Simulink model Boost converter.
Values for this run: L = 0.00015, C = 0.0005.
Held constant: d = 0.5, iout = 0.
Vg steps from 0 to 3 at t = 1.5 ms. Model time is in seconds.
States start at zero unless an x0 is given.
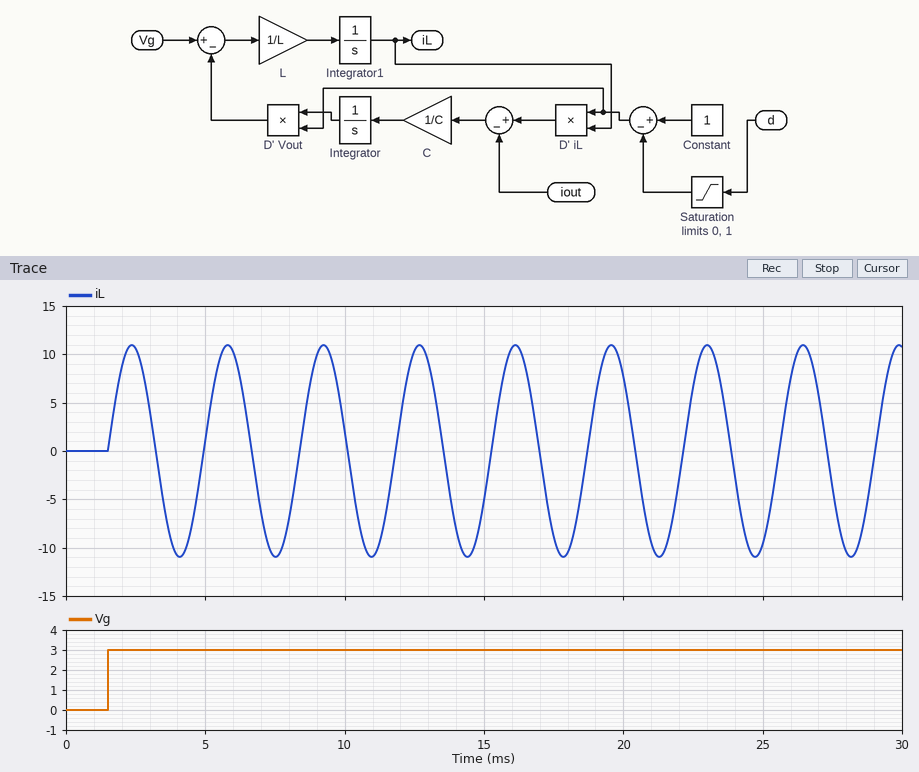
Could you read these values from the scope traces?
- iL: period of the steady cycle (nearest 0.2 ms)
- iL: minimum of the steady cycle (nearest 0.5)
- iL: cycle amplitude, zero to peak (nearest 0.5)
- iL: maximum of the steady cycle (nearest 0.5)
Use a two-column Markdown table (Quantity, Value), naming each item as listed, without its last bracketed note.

| Quantity | Value |
|---|---|
| iL: period of the steady cycle | 3.4 ms |
| iL: minimum of the steady cycle | -11.0 |
| iL: cycle amplitude, zero to peak | 11.0 |
| iL: maximum of the steady cycle | 11.0 |
